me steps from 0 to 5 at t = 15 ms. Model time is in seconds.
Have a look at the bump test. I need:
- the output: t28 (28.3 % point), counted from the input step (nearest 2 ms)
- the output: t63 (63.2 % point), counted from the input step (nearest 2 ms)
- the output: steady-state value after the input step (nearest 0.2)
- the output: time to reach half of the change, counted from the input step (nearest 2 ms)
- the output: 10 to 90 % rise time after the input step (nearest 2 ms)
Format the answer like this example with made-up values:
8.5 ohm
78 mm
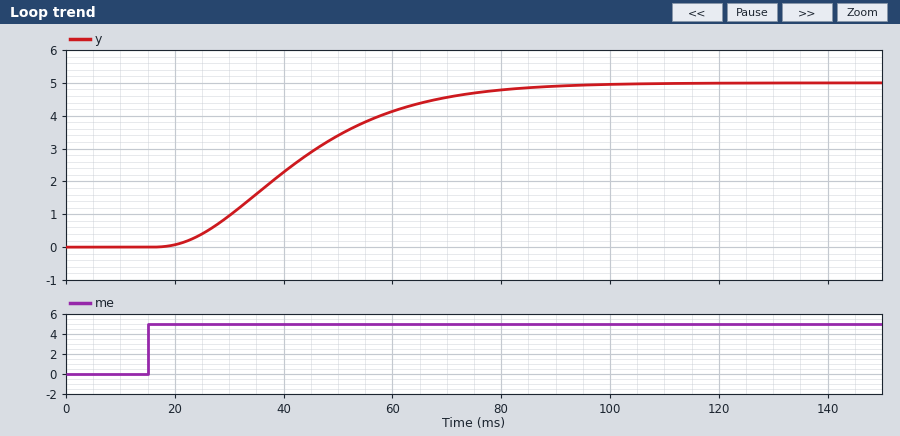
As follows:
18 ms
32 ms
5.0
26 ms
42 ms
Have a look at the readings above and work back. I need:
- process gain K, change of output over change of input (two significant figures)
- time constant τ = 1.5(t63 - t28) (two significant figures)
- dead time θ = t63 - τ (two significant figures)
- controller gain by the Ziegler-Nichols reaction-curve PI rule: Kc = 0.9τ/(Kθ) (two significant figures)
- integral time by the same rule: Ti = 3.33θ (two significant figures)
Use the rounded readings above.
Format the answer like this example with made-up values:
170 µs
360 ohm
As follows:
1.0
21 ms
11 ms
1.7
37 ms
